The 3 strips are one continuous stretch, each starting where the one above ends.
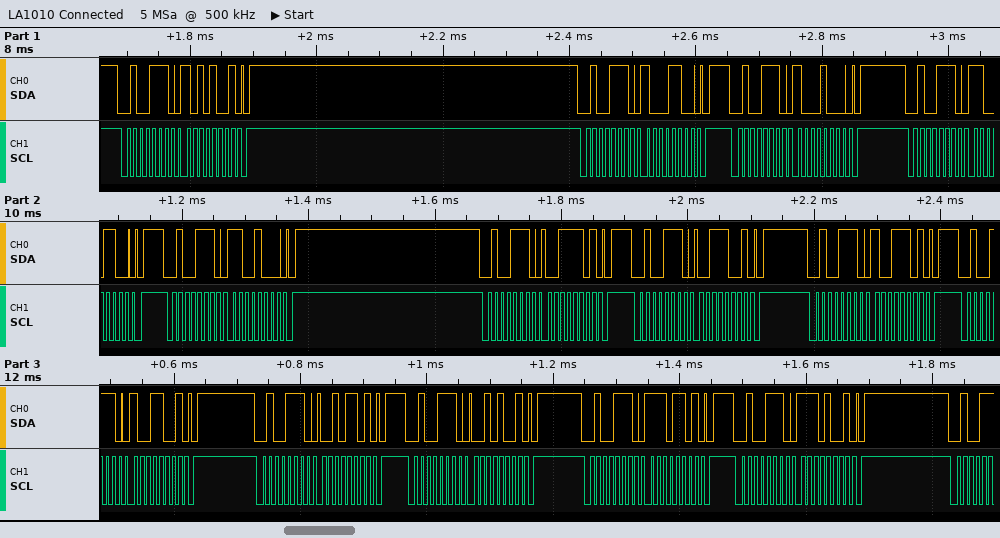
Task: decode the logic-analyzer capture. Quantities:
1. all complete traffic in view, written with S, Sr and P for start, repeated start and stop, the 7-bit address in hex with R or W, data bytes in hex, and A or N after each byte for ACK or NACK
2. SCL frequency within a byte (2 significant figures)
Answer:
S 27W A A9 A P S 27W A 8C A P S 27W A 88 A P S 27W A CC A P S 27W A C8 A P S 27W A 3D A P S 27W A 39 A P S 27W A 9D A P S 27W A 99 A P S 27W A 2D A P S 27W A 29 A P S 27W A ED A P S 27W A E9 A P
100 kHz
